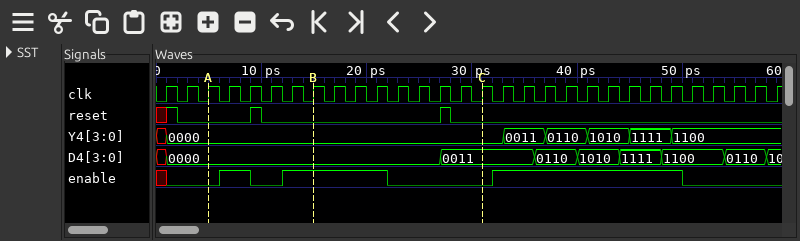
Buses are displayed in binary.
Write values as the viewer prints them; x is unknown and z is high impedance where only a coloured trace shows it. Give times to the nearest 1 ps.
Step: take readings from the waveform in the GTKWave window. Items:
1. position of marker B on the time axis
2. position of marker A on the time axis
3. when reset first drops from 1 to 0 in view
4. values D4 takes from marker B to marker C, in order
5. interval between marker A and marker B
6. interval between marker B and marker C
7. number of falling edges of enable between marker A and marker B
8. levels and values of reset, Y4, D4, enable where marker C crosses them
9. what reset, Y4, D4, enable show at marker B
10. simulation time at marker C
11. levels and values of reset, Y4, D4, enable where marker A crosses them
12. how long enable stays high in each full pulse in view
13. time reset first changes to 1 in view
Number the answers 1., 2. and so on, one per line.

1. 15 ps
2. 5 ps
3. 2 ps
4. 0000, 0011
5. 10 ps
6. 16 ps
7. 1
8. reset=0, Y4=0000, D4=0011, enable=0
9. reset=0, Y4=0000, D4=0000, enable=1
10. 31 ps
11. reset=0, Y4=0000, D4=0000, enable=0
12. 3 ps, 10 ps, 18 ps
13. 1 ps
